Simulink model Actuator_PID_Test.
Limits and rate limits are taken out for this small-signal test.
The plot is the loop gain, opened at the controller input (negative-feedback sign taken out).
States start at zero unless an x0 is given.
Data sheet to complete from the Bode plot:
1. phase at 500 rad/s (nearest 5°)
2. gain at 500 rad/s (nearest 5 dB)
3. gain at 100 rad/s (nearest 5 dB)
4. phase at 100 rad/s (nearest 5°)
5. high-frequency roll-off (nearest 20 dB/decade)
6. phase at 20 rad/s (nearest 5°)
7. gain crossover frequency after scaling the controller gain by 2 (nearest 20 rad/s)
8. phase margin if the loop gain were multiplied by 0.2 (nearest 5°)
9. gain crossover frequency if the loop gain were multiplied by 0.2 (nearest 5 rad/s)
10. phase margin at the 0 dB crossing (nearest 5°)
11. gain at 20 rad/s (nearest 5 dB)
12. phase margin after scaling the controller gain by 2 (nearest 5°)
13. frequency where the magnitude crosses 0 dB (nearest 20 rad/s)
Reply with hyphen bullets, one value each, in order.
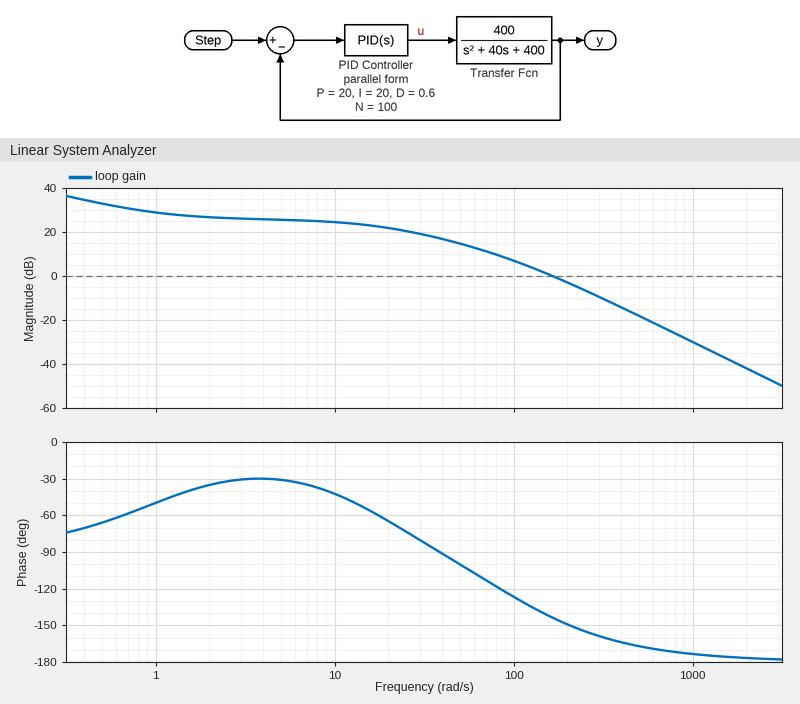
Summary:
- -165°
- -20 dB
- 5 dB
- -125°
- -40 dB/decade
- -65°
- 240 rad/s
- 75°
- 55 rad/s
- 35°
- 20 dB
- 25°
- 160 rad/s
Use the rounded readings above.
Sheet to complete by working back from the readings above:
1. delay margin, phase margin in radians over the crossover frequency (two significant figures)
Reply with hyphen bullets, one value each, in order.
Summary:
- 0.0038 s
